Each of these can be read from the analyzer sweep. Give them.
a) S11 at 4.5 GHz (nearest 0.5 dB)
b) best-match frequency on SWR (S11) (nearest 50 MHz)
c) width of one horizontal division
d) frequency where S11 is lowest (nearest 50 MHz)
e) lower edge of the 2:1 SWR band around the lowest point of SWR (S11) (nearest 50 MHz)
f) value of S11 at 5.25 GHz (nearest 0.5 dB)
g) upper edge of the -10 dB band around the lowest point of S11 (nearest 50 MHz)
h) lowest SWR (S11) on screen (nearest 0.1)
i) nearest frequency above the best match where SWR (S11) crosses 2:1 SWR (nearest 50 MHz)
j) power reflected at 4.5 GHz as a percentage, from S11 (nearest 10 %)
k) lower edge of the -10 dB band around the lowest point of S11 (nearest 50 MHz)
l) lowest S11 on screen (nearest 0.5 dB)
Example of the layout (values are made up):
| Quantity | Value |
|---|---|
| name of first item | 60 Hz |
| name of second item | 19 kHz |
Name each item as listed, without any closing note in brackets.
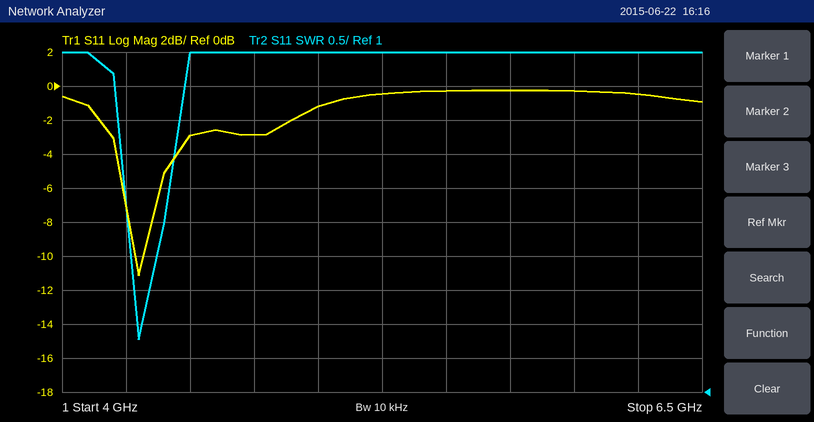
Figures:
| Quantity | Value |
|---|---|
| S11 at 4.5 GHz | -3.0 dB |
| best-match frequency on SWR (S11) | 4.30 GHz |
| width of one horizontal division | 250 MHz |
| frequency where S11 is lowest | 4.30 GHz |
| lower edge of the 2:1 SWR band around the lowest point of SWR (S11) | 4.30 GHz |
| value of S11 at 5.25 GHz | -0.5 dB |
| upper edge of the -10 dB band around the lowest point of S11 | 4.30 GHz |
| lowest SWR (S11) on screen | 1.8 |
| nearest frequency above the best match where SWR (S11) crosses 2:1 SWR | 4.30 GHz |
| power reflected at 4.5 GHz as a percentage, from S11 | 50 % |
| lower edge of the -10 dB band around the lowest point of S11 | 4.30 GHz |
| lowest S11 on screen | -11.0 dB |
